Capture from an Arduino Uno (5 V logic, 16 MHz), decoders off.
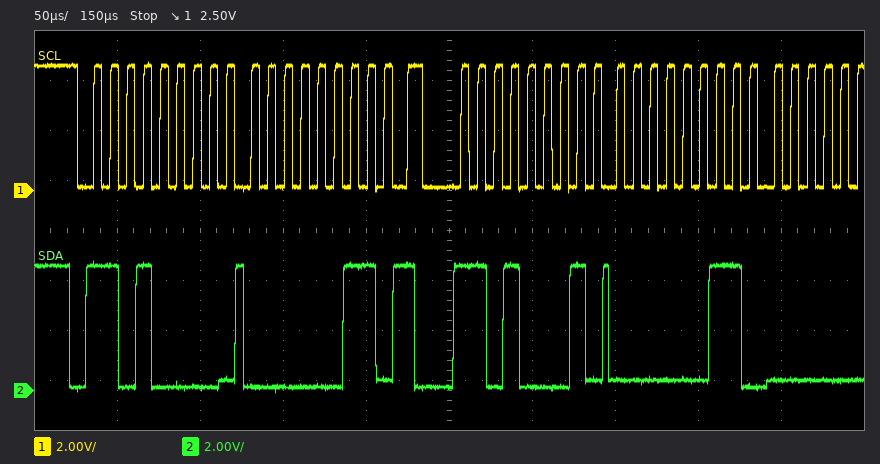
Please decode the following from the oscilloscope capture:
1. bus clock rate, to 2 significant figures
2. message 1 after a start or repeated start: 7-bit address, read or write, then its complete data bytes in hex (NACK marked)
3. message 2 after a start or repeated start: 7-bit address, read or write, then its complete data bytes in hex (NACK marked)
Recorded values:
100 kHz
0x68 write: 03
0x68 read: 03
